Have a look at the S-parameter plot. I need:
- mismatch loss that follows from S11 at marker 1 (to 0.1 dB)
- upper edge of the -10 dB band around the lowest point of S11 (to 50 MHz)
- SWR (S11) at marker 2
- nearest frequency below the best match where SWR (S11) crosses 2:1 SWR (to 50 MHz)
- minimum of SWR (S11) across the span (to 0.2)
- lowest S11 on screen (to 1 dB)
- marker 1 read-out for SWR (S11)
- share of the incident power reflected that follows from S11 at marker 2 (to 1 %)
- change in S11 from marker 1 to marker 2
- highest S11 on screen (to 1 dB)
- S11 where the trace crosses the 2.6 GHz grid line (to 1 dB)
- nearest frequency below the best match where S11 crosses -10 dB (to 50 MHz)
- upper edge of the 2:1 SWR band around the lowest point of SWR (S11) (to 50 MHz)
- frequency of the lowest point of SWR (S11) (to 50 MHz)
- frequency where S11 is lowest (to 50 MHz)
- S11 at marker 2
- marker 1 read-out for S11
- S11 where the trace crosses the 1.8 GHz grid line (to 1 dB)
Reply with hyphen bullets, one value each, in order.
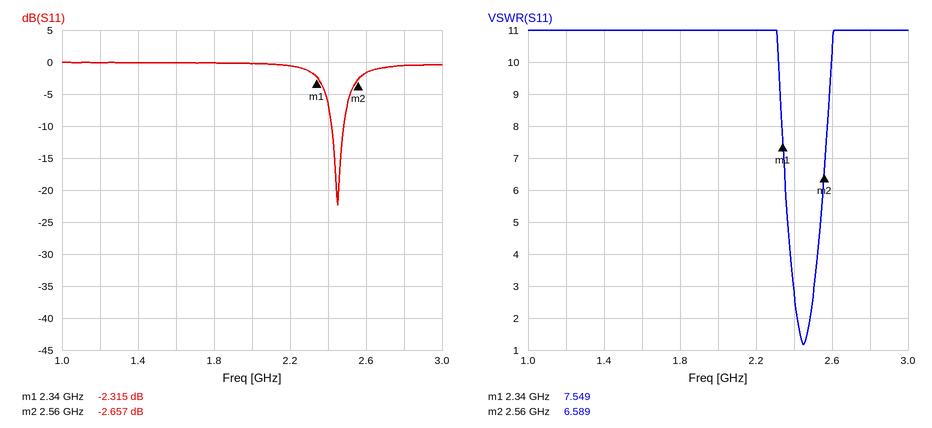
- 3.8 dB
- 2.50 GHz
- 6.589
- 2.40 GHz
- 1.2
- -22 dB
- 7.549
- 54 %
- -0.342 dB
- 0 dB
- -2 dB
- 2.40 GHz
- 2.50 GHz
- 2.45 GHz
- 2.45 GHz
- -2.657 dB
- -2.315 dB
- 0 dB
